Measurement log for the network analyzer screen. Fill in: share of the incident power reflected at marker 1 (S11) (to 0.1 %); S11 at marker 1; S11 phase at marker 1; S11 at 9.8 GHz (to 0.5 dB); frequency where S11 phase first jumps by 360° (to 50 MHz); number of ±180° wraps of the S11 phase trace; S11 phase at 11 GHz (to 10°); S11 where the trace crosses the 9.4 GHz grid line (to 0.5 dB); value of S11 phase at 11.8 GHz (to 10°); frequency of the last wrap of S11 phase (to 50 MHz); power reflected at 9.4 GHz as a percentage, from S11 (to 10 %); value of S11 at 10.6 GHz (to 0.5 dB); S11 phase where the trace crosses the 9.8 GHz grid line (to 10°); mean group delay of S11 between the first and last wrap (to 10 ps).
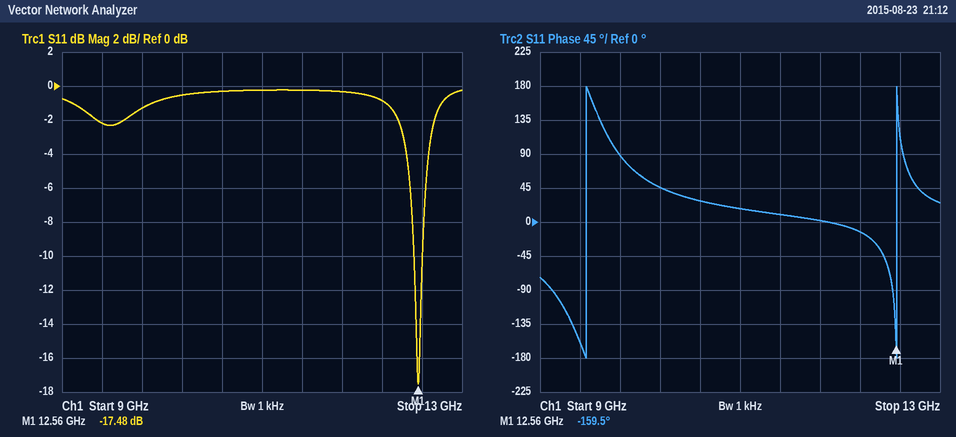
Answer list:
1.8 %
-17.48 dB
-159.5°
-1.5 dB
9.45 GHz
2
20°
-2.0 dB
0°
12.55 GHz
60 %
-0.5 dB
90°
320 ps
